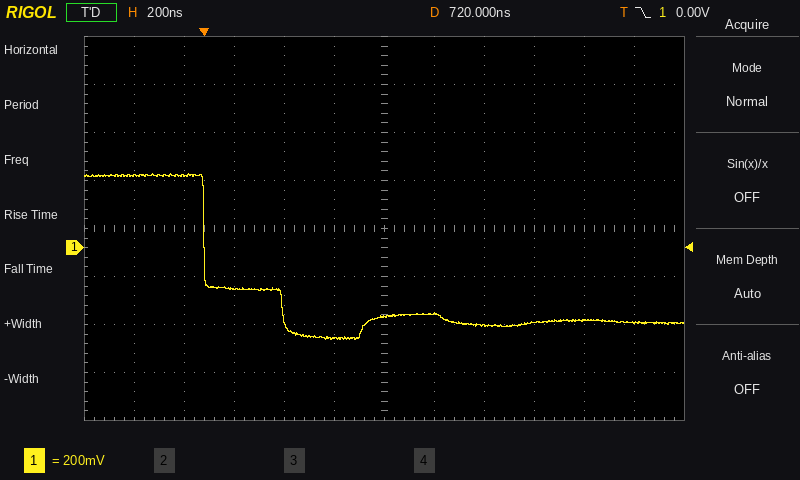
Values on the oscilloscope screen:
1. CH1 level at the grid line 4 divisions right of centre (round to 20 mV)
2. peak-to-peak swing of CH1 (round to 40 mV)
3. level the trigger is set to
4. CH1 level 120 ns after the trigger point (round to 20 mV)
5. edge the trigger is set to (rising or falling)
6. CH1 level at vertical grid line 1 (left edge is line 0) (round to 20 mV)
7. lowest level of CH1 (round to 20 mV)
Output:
-300 mV
680 mV
0.00 V
-180 mV
falling
300 mV
-380 mV
